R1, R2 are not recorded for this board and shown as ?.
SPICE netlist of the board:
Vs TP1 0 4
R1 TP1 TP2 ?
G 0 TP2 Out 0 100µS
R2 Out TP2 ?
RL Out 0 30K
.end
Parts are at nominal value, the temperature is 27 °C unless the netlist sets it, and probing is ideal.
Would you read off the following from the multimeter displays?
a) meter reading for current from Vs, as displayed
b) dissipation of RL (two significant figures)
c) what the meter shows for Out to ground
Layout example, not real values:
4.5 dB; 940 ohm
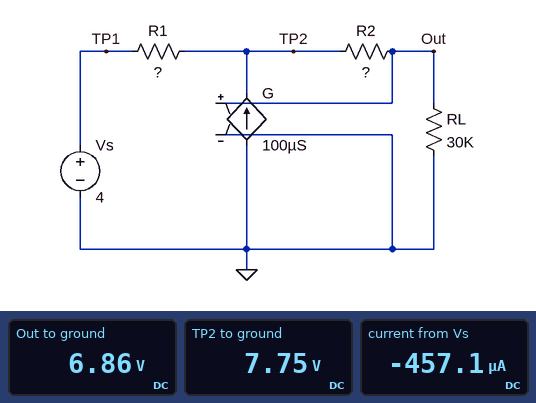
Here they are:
-457.1 µA; 1.6 mW; 6.86 V
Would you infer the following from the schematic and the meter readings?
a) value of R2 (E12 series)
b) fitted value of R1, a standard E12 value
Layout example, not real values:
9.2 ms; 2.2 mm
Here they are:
3.9 kΩ; 8.2 kΩ
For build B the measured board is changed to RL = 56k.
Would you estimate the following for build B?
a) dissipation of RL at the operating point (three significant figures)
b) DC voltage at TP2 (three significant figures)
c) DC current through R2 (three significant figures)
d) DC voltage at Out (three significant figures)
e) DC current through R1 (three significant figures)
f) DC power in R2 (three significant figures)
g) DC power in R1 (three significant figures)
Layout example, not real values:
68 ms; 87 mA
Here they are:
1.82 mW; 10.8 V; 180 µA; 10.1 V; 830 µA; 127 µW; 5.64 mW
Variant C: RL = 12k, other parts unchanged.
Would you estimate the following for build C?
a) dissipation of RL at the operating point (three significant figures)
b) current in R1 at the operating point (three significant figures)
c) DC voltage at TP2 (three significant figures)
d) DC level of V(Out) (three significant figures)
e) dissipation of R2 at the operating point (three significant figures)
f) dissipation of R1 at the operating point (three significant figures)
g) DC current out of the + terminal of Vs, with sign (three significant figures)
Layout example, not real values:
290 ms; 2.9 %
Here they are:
944 µW; 56.1 µA; 4.46 V; 3.37 V; 307 µW; 25.8 µW; -56.1 µA
